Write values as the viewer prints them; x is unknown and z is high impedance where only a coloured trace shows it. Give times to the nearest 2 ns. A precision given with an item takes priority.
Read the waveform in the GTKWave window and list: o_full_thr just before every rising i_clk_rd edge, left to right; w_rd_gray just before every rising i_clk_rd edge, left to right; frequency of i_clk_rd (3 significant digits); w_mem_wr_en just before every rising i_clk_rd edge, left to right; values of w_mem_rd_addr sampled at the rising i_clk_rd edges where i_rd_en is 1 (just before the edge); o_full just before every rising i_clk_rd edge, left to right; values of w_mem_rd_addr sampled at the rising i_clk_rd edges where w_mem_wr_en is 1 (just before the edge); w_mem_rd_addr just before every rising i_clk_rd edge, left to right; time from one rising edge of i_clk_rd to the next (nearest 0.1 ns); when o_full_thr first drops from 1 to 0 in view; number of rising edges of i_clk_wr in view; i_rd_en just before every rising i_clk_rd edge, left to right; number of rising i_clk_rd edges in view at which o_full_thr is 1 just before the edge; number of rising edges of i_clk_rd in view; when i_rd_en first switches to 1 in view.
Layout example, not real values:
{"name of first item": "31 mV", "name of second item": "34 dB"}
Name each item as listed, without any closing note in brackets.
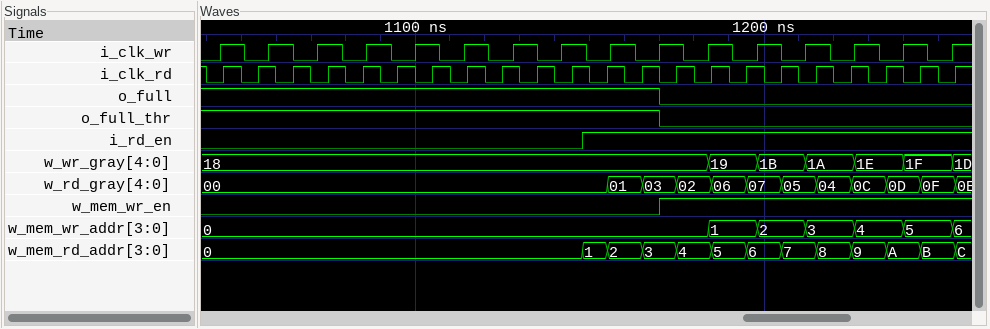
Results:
{"o_full_thr just before every rising i_clk_rd edge, left to right": "1 1 1 1 1 1 1 1 1 1 1 1 1 0 0 0 0 0 0 0 0 0", "w_rd_gray just before every rising i_clk_rd edge, left to right": "00, 00, 00, 00, 00, 00, 00, 00, 00, 00, 00, 00, 01, 03, 02, 06, 07, 05, 04, 0C, 0D, 0F", "frequency of i_clk_rd": "100 MHz", "w_mem_wr_en just before every rising i_clk_rd edge, left to right": "0 0 0 0 0 0 0 0 0 0 0 0 0 1 1 1 1 1 1 1 1 1", "values of w_mem_rd_addr sampled at the rising i_clk_rd edges where i_rd_en is 1": "1, 2, 3, 4, 5, 6, 7, 8, 9, A, B", "o_full just before every rising i_clk_rd edge, left to right": "1 1 1 1 1 1 1 1 1 1 1 1 1 0 0 0 0 0 0 0 0 0", "values of w_mem_rd_addr sampled at the rising i_clk_rd edges where w_mem_wr_en is 1": "3, 4, 5, 6, 7, 8, 9, A, B", "w_mem_rd_addr just before every rising i_clk_rd edge, left to right": "0, 0, 0, 0, 0, 0, 0, 0, 0, 0, 0, 1, 2, 3, 4, 5, 6, 7, 8, 9, A, B", "time from one rising edge of i_clk_rd to the next": "10 ns", "when o_full_thr first drops from 1 to 0 in view": "1170 ns", "number of rising edges of i_clk_wr in view": "16", "i_rd_en just before every rising i_clk_rd edge, left to right": "0 0 0 0 0 0 0 0 0 0 0 1 1 1 1 1 1 1 1 1 1 1", "number of rising i_clk_rd edges in view at which o_full_thr is 1 just before the edge": "13", "number of rising edges of i_clk_rd in view": "22", "when i_rd_en first switches to 1 in view": "1148 ns"}
